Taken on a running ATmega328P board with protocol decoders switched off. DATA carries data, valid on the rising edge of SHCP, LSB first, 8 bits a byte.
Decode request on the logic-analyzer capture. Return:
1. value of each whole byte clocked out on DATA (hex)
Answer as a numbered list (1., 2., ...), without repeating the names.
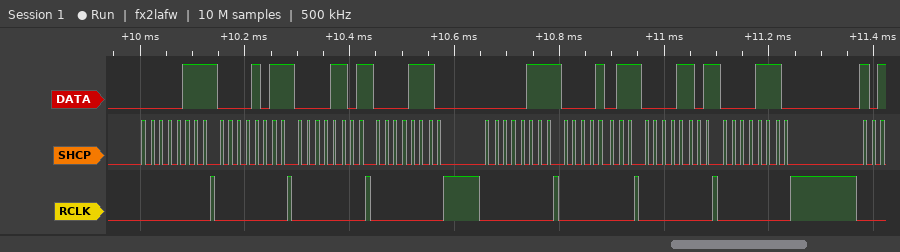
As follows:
1. E0 D0 B0 70 E0 D0 B0 70
